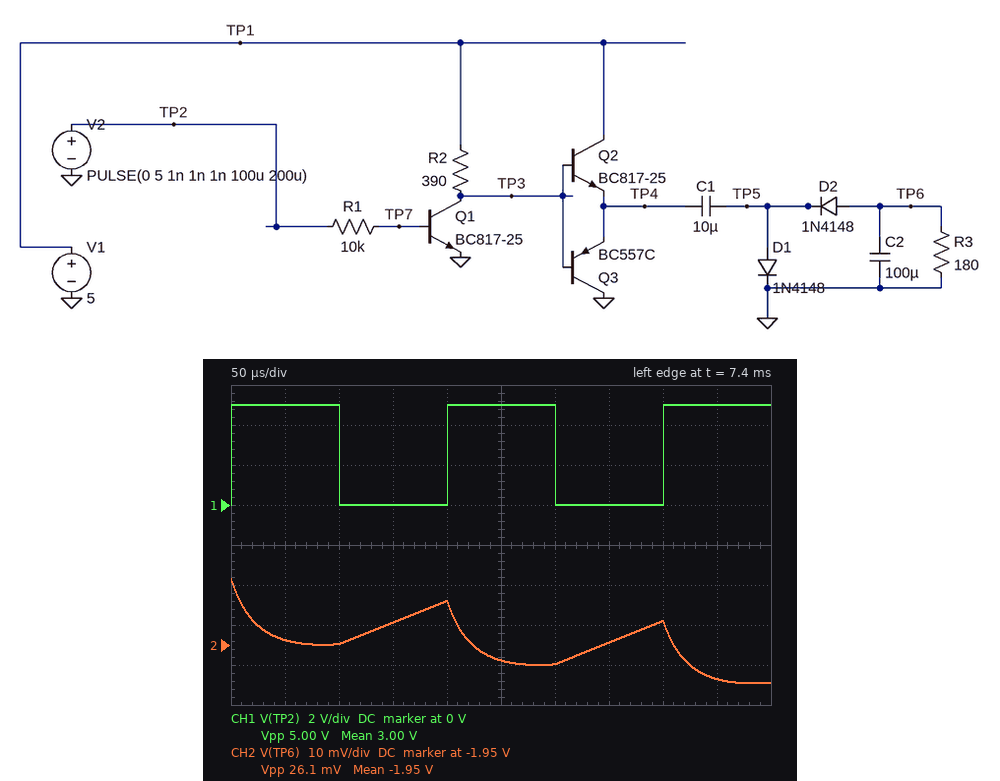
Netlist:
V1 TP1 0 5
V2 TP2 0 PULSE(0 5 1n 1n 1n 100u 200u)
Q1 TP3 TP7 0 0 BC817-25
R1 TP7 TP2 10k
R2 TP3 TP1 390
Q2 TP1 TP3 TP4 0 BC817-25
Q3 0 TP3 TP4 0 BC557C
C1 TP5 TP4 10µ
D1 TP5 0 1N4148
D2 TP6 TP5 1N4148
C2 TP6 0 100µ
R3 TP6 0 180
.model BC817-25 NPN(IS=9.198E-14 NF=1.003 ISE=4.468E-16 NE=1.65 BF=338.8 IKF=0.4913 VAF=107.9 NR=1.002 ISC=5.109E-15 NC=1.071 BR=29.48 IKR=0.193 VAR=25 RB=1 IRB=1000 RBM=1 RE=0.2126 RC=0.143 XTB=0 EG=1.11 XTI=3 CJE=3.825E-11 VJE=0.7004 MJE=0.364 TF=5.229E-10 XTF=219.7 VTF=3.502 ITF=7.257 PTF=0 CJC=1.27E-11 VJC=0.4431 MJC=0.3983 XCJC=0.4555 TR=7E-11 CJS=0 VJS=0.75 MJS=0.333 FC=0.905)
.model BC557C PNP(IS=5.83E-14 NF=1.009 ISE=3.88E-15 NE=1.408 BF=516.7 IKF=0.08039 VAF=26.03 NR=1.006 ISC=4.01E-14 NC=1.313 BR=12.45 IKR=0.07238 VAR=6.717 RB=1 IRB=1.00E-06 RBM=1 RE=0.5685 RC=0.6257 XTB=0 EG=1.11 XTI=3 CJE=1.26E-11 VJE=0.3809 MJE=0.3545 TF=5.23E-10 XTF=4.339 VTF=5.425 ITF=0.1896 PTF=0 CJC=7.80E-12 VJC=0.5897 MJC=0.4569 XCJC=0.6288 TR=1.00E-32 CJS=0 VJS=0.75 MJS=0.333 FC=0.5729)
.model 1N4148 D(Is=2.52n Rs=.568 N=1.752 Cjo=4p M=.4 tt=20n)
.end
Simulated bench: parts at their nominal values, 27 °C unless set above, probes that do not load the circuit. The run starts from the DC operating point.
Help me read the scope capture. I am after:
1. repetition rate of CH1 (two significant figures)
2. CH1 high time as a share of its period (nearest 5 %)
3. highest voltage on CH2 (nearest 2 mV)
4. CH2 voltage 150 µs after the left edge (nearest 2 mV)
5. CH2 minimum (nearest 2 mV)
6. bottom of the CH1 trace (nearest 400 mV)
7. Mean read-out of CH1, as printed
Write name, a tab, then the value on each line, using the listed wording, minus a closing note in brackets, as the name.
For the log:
repetition rate of CH1	5.0 kHz
CH1 high time as a share of its period	50 %
highest voltage on CH2	-1.934 V
CH2 voltage 150 µs after the left edge	-1.944 V
CH2 minimum	-1.960 V
bottom of the CH1 trace	0 V
Mean read-out of CH1, as printed	3.00 V
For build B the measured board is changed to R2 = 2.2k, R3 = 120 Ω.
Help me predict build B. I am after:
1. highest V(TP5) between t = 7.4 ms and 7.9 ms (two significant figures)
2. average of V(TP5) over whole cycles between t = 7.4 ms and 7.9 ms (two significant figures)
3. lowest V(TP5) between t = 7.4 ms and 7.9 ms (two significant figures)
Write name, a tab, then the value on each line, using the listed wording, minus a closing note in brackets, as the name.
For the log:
highest V(TP5) between t = 7.4 ms and 7.9 ms	800 mV
average of V(TP5) over whole cycles between t = 7.4 ms and 7.9 ms	-840 mV
lowest V(TP5) between t = 7.4 ms and 7.9 ms	-2.6 V
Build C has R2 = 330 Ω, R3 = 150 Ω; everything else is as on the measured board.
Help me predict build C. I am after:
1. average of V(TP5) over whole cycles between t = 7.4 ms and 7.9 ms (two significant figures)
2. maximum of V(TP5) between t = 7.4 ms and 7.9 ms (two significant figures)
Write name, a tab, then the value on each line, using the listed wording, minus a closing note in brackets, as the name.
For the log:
average of V(TP5) over whole cycles between t = 7.4 ms and 7.9 ms	-960 mV
maximum of V(TP5) between t = 7.4 ms and 7.9 ms	830 mV
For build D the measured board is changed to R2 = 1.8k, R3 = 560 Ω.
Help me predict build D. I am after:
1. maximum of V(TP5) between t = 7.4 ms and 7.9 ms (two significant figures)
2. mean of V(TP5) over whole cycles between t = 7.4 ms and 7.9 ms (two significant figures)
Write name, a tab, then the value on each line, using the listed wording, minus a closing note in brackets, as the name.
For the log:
maximum of V(TP5) between t = 7.4 ms and 7.9 ms	760 mV
mean of V(TP5) over whole cycles between t = 7.4 ms and 7.9 ms	-1.0 V
